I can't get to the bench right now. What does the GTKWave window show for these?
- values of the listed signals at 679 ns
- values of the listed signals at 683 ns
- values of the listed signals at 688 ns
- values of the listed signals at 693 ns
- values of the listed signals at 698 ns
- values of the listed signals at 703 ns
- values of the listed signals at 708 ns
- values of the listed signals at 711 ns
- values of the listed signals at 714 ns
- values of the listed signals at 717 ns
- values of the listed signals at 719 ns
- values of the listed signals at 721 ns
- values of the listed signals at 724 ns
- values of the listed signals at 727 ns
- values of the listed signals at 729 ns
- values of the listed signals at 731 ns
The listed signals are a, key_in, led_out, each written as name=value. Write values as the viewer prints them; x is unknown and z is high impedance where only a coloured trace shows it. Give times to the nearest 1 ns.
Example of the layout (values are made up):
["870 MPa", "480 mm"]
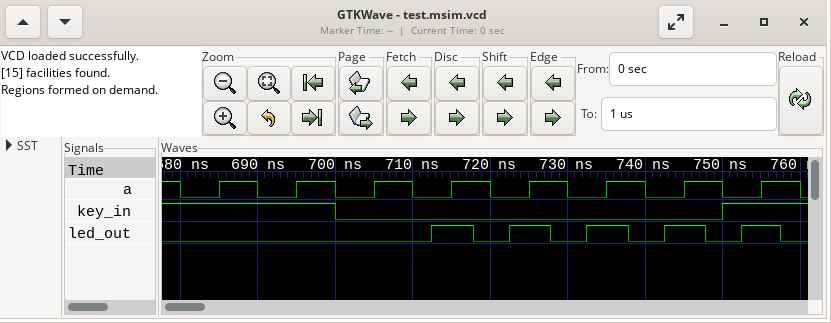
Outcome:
["a=1, key_in=1, led_out=0", "a=0, key_in=1, led_out=0", "a=1, key_in=1, led_out=0", "a=0, key_in=1, led_out=0", "a=1, key_in=1, led_out=0", "a=0, key_in=0, led_out=0", "a=1, key_in=0, led_out=0", "a=0, key_in=0, led_out=0", "a=0, key_in=0, led_out=1", "a=1, key_in=0, led_out=1", "a=1, key_in=0, led_out=0", "a=0, key_in=0, led_out=0", "a=0, key_in=0, led_out=1", "a=1, key_in=0, led_out=1", "a=1, key_in=0, led_out=0", "a=0, key_in=0, led_out=0"]
